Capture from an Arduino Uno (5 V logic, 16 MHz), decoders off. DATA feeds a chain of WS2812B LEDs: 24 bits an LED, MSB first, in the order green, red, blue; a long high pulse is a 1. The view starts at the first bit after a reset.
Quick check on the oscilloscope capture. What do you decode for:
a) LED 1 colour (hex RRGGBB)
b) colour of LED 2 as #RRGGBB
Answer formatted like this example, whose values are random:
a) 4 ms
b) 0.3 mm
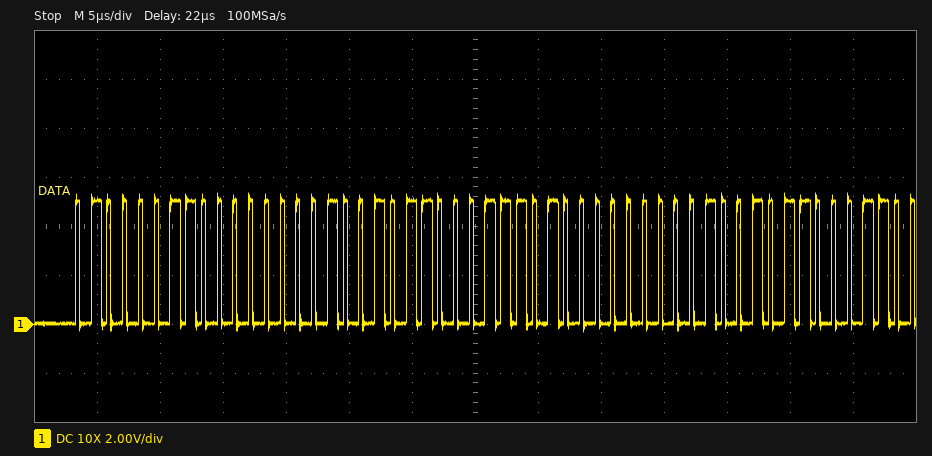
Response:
a) #004396
b) #003A96
